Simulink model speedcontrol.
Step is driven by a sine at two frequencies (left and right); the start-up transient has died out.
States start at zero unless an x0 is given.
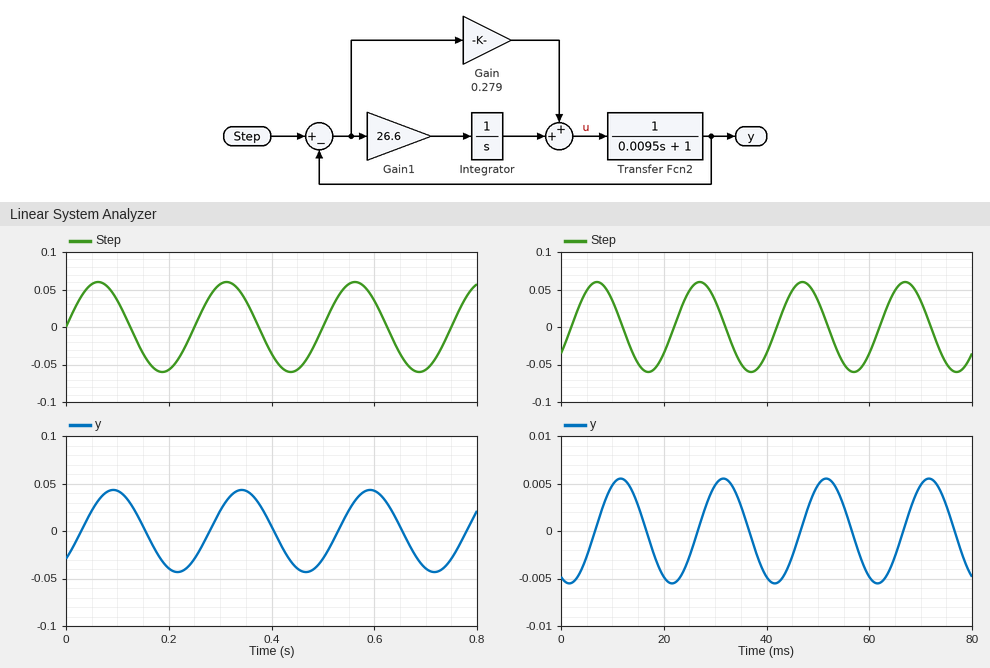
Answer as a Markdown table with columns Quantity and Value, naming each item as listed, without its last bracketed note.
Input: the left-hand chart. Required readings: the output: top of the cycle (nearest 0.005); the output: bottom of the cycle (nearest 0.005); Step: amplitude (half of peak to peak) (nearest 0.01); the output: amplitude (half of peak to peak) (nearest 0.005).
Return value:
| Quantity | Value |
|---|---|
| the output: top of the cycle | 0.045 |
| the output: bottom of the cycle | -0.045 |
| Step: amplitude (half of peak to peak) | 0.06 |
| the output: amplitude (half of peak to peak) | 0.045 |
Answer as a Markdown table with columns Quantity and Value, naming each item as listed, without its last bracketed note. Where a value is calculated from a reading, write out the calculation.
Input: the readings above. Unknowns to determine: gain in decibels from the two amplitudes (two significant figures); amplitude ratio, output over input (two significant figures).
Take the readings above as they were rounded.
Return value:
| Quantity | Value |
|---|---|
| gain in decibels from the two amplitudes | 20 log10(0.045 / 0.06) = -2.5 dB |
| amplitude ratio, output over input | 0.045 / 0.06 = 0.75 |
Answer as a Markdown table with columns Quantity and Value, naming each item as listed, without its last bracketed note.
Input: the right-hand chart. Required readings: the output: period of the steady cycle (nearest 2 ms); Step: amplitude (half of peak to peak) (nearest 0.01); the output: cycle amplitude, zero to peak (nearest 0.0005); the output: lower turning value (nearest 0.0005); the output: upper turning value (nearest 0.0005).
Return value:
| Quantity | Value |
|---|---|
| the output: period of the steady cycle | 20 ms |
| Step: amplitude (half of peak to peak) | 0.06 |
| the output: cycle amplitude, zero to peak | 0.0055 |
| the output: lower turning value | -0.0055 |
| the output: upper turning value | 0.0055 |
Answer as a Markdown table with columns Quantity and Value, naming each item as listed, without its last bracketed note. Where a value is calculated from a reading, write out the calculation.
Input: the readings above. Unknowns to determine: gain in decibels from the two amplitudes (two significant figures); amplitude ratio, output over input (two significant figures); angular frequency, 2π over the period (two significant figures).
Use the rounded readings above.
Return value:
| Quantity | Value |
|---|---|
| gain in decibels from the two amplitudes | 20 log10(0.0055 / 0.06) = -21 dB |
| amplitude ratio, output over input | 0.0055 / 0.06 = 0.092 |
| angular frequency, 2π over the period | 2π / 20 = 0.31 rad/ms |
